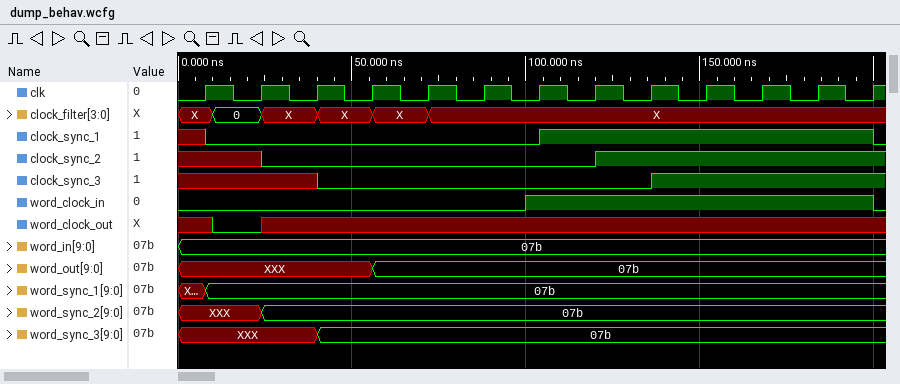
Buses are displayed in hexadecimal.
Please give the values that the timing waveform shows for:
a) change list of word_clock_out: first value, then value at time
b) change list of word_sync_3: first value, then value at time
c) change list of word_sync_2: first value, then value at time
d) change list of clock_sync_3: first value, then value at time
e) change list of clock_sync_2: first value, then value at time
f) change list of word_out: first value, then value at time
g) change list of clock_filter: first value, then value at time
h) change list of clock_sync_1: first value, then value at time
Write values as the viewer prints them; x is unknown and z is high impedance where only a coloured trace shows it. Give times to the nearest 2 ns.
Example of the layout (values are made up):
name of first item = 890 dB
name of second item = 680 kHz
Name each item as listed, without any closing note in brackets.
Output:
change list of word_clock_out: first value, then value at time = x, 0 at 10 ns, x at 24 ns
change list of word_sync_3: first value, then value at time = XXX, 07b at 40 ns
change list of word_sync_2: first value, then value at time = XXX, 07b at 24 ns
change list of clock_sync_3: first value, then value at time = x, 0 at 40 ns, 1 at 136 ns
change list of clock_sync_2: first value, then value at time = x, 0 at 24 ns, 1 at 120 ns
change list of word_out: first value, then value at time = XXX, 07b at 56 ns
change list of clock_filter: first value, then value at time = X, 0 at 10 ns, X at 24 ns, X at 40 ns, X at 56 ns, X at 72 ns
change list of clock_sync_1: first value, then value at time = x, 0 at 8 ns, 1 at 104 ns, 0 at 200 ns
